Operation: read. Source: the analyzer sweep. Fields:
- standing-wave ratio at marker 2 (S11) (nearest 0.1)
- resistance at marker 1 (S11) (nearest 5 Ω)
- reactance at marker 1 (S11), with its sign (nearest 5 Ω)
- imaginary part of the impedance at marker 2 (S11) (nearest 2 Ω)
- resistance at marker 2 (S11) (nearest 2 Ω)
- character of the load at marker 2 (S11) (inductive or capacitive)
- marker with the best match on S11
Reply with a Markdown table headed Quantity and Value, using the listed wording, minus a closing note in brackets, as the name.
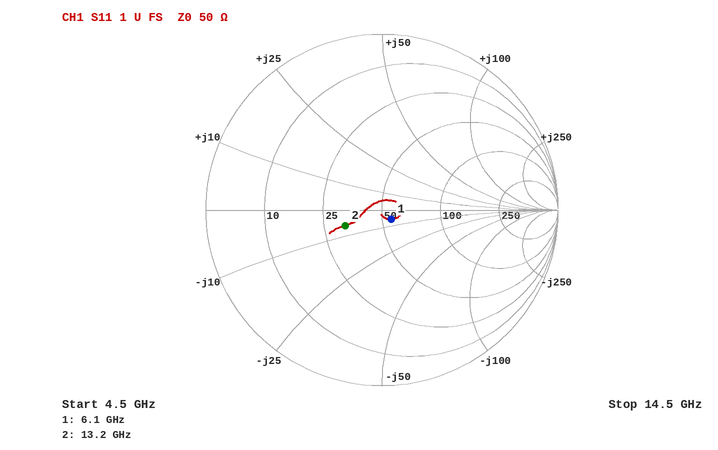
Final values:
| Quantity | Value |
|---|---|
| standing-wave ratio at marker 2 (S11) | 1.6 |
| resistance at marker 1 (S11) | 55 Ω |
| reactance at marker 1 (S11), with its sign | -5 Ω |
| imaginary part of the impedance at marker 2 (S11) | -6 Ω |
| resistance at marker 2 (S11) | 32 Ω |
| character of the load at marker 2 (S11) | capacitive |
| marker with the best match on S11 | marker 1 |
